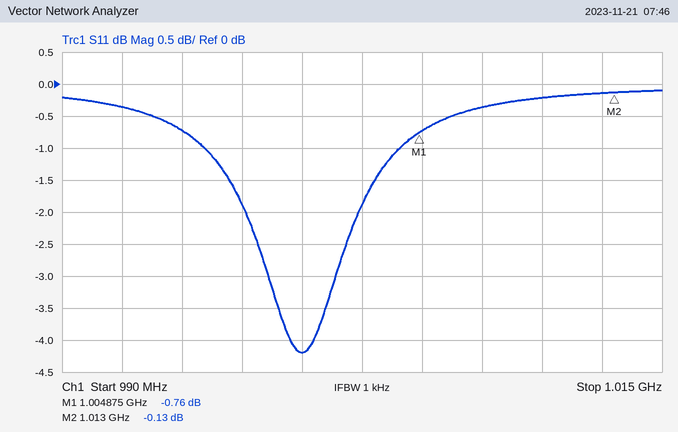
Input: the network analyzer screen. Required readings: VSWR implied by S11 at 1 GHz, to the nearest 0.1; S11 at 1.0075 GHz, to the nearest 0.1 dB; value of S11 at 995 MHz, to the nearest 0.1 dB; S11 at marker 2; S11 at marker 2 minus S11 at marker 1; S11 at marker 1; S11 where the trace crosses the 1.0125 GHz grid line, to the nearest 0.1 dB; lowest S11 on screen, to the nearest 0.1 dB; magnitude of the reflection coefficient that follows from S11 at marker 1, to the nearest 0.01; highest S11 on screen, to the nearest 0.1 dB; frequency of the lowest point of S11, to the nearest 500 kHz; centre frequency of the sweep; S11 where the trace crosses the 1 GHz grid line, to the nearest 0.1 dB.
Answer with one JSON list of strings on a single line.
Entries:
["4.2", "-0.4 dB", "-0.7 dB", "-0.13 dB", "0.63 dB", "-0.76 dB", "-0.1 dB", "-4.2 dB", "0.92", "-0.1 dB", "1.0000 GHz", "1.0025 GHz", "-4.2 dB"]
